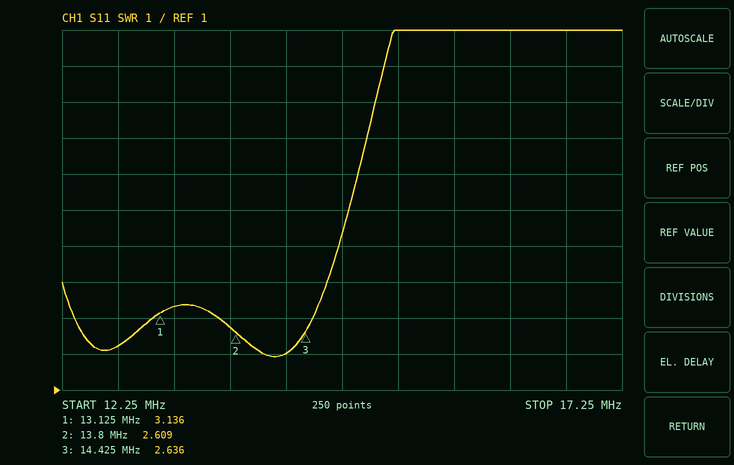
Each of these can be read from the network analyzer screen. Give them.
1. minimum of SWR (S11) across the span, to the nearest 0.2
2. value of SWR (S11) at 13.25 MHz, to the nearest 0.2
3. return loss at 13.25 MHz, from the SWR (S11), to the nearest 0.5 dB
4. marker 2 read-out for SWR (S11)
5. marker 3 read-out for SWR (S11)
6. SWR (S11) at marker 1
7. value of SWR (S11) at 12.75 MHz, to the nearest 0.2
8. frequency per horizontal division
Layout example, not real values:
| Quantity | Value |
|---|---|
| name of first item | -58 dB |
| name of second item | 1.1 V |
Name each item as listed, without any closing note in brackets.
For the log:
| Quantity | Value |
|---|---|
| minimum of SWR (S11) across the span, to the nearest 0.2 | 2.0 |
| value of SWR (S11) at 13.25 MHz, to the nearest 0.2 | 3.4 |
| return loss at 13.25 MHz, from the SWR (S11), to the nearest 0.5 dB | 5.5 dB |
| marker 2 read-out for SWR | 2.609 |
| marker 3 read-out for SWR | 2.636 |
| SWR (S11) at marker 1 | 3.136 |
| value of SWR (S11) at 12.75 MHz, to the nearest 0.2 | 2.2 |
| frequency per horizontal division | 500 kHz |
